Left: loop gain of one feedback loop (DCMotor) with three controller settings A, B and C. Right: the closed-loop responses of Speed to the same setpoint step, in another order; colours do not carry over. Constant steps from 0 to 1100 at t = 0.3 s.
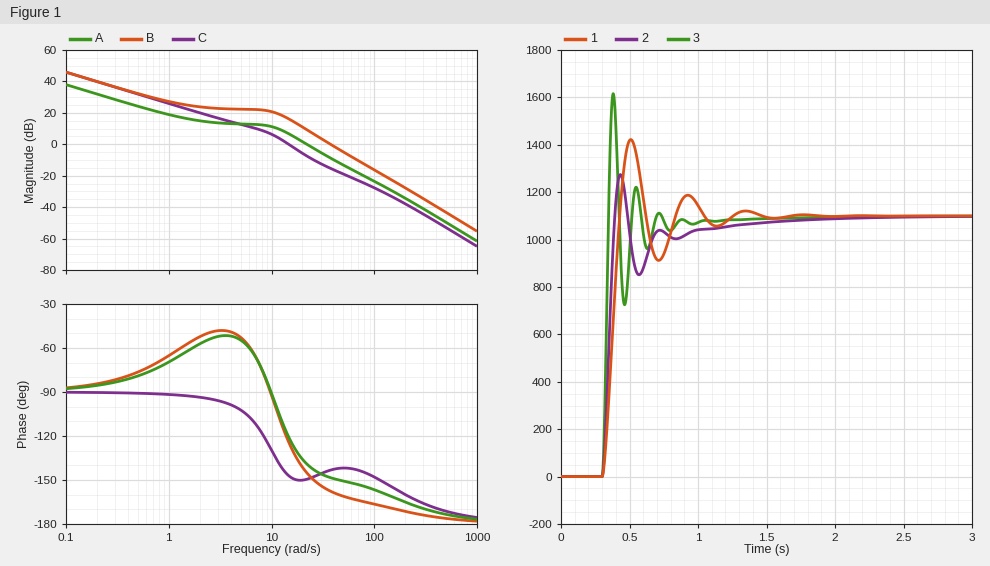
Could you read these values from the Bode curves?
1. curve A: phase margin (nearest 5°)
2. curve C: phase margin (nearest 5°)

40°
35°
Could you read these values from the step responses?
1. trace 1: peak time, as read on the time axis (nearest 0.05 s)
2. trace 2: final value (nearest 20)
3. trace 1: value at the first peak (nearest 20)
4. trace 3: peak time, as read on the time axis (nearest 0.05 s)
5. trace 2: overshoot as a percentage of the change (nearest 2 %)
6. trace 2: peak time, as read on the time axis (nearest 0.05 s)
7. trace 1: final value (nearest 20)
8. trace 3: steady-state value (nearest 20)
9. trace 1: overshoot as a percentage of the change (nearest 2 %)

0.50 s
1100
1420
0.40 s
16 %
0.45 s
1100
1100
30 %
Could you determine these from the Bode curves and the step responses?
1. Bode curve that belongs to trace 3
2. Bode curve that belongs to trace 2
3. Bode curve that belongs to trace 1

B
A
C
